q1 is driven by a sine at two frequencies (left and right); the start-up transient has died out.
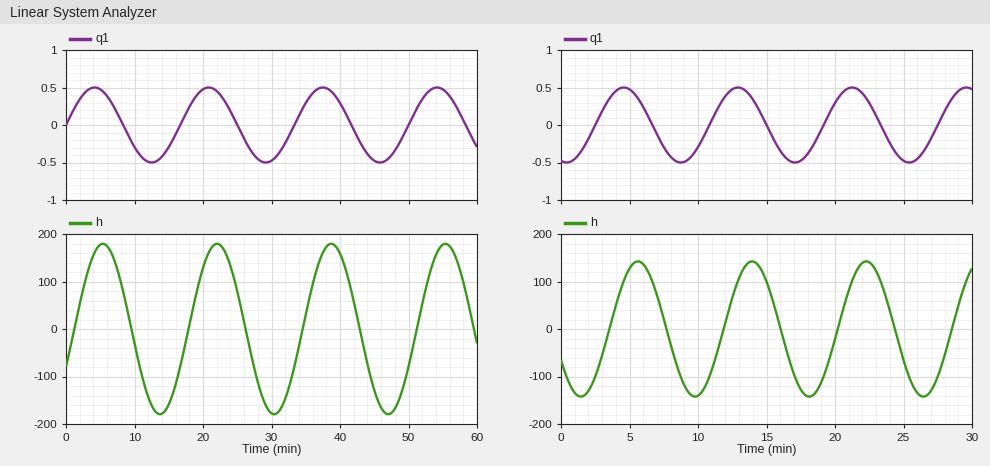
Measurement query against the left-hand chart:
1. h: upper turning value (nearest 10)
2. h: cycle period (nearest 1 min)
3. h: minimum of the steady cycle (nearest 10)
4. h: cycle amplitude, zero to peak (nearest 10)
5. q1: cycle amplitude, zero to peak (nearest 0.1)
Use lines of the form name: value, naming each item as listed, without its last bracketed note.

h: upper turning value: 180
h: cycle period: 17 min
h: minimum of the steady cycle: -180
h: cycle amplitude, zero to peak: 180
q1: cycle amplitude, zero to peak: 0.5
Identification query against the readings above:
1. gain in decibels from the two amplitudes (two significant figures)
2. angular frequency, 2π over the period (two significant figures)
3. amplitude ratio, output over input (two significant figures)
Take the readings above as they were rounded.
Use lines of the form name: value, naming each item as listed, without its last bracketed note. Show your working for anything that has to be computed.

gain in decibels from the two amplitudes: 20 log10(180 / 0.5) = 51 dB
angular frequency, 2π over the period: 2π / 17 = 0.37 rad/min
amplitude ratio, output over input: 180 / 0.5 = 360
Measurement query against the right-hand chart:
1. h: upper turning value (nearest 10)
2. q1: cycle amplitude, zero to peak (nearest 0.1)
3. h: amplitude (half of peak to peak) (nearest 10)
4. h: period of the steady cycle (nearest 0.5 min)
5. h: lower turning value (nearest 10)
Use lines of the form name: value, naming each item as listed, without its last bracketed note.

h: upper turning value: 140
q1: cycle amplitude, zero to peak: 0.5
h: amplitude (half of peak to peak): 140
h: period of the steady cycle: 8.5 min
h: lower turning value: -140
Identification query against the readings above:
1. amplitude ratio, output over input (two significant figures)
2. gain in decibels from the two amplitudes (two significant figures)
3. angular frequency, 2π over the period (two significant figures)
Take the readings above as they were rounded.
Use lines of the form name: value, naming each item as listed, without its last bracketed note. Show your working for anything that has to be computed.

amplitude ratio, output over input: 140 / 0.5 = 280
gain in decibels from the two amplitudes: 20 log10(140 / 0.5) = 49 dB
angular frequency, 2π over the period: 2π / 8.5 = 0.74 rad/min
